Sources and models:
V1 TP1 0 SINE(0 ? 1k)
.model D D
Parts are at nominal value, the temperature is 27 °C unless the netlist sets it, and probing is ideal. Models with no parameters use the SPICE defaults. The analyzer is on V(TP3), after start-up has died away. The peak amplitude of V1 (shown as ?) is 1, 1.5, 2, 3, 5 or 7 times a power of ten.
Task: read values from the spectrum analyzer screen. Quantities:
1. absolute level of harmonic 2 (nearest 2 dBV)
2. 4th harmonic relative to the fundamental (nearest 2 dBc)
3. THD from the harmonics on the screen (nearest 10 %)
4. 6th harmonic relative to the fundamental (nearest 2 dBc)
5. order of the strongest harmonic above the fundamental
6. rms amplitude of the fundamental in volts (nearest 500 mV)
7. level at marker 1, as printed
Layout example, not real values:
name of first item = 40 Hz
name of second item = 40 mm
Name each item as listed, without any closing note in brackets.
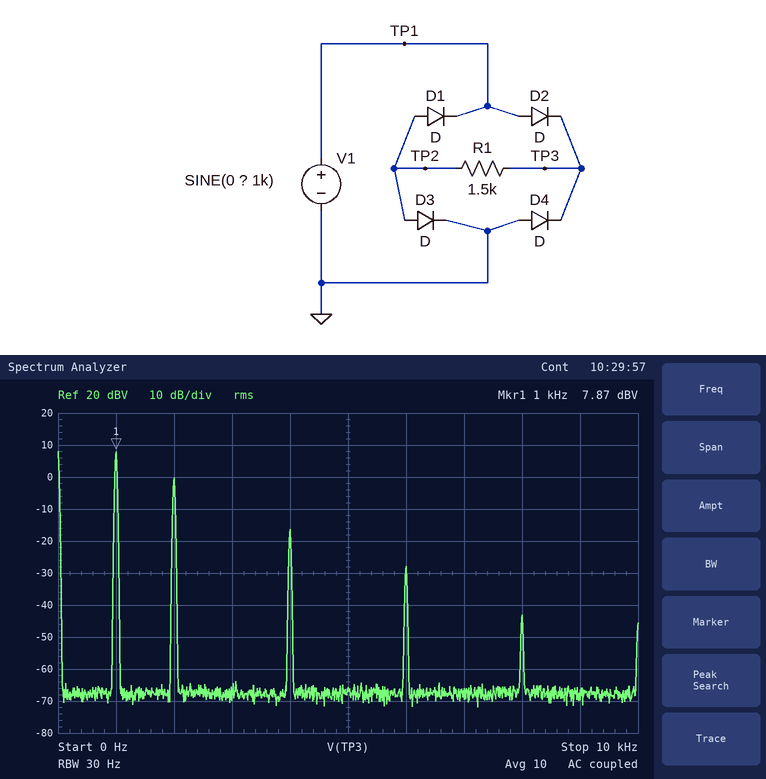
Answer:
absolute level of harmonic 2 = 0 dBV
4th harmonic relative to the fundamental = -24 dBc
THD from the harmonics on the screen = 40 %
6th harmonic relative to the fundamental = -36 dBc
order of the strongest harmonic above the fundamental = 2
rms amplitude of the fundamental in volts = 2.5 V
level at marker 1, as printed = 7.87 dBV
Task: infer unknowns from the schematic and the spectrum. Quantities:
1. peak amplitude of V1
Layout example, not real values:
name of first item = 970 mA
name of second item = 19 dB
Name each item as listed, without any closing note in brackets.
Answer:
peak amplitude of V1 = 7 V
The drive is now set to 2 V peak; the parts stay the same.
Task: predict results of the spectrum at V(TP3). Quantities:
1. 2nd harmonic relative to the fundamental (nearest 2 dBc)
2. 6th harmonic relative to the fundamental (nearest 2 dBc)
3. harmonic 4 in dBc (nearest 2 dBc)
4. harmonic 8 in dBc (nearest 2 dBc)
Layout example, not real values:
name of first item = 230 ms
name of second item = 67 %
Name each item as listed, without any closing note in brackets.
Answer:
2nd harmonic relative to the fundamental = -14 dBc
6th harmonic relative to the fundamental = -34 dBc
harmonic 4 in dBc = -28 dBc
harmonic 8 in dBc = -54 dBc
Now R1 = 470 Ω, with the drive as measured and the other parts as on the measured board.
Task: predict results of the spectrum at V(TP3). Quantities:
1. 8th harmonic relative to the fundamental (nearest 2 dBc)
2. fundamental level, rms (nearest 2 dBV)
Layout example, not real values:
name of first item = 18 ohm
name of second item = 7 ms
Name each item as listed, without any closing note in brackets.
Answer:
8th harmonic relative to the fundamental = -56 dBc
fundamental level, rms = 8 dBV
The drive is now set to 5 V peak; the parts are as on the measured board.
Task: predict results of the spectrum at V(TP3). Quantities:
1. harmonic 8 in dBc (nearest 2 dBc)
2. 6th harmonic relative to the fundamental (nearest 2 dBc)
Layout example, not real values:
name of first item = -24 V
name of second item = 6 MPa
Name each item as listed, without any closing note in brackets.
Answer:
harmonic 8 in dBc = -44 dBc
6th harmonic relative to the fundamental = -50 dBc
